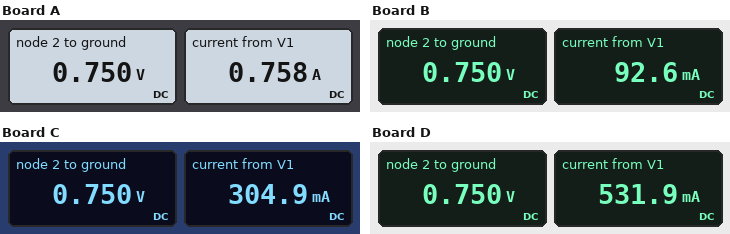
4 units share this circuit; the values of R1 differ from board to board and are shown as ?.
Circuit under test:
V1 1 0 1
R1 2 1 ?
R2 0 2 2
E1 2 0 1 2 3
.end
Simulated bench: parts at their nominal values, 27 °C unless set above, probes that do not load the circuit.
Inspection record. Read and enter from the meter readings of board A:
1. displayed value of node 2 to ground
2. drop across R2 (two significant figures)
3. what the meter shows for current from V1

0.750 V
750 mV
0.758 A
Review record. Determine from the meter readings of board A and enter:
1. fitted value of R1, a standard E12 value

0.33 Ω
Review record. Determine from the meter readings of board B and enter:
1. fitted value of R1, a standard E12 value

2.7 Ω
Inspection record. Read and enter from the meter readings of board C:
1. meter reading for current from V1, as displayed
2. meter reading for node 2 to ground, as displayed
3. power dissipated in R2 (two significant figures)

304.9 mA
0.750 V
280 mW
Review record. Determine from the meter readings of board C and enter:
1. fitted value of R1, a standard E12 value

0.82 Ω
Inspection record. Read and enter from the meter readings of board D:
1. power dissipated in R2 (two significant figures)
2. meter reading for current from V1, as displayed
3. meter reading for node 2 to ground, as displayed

280 mW
531.9 mA
0.750 V
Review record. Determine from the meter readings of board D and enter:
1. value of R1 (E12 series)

0.47 Ω
